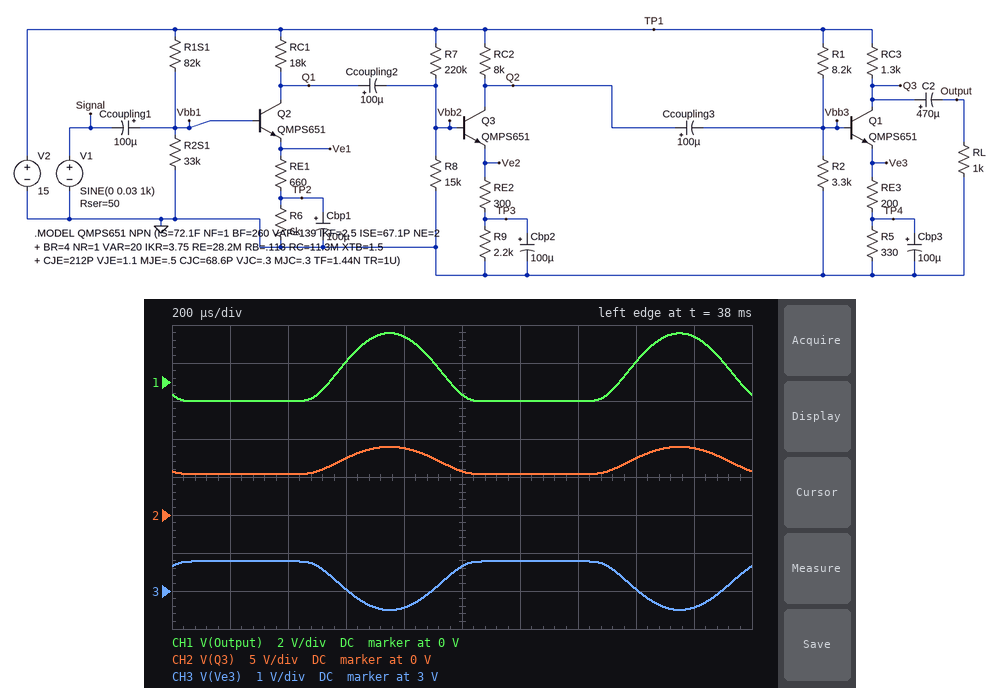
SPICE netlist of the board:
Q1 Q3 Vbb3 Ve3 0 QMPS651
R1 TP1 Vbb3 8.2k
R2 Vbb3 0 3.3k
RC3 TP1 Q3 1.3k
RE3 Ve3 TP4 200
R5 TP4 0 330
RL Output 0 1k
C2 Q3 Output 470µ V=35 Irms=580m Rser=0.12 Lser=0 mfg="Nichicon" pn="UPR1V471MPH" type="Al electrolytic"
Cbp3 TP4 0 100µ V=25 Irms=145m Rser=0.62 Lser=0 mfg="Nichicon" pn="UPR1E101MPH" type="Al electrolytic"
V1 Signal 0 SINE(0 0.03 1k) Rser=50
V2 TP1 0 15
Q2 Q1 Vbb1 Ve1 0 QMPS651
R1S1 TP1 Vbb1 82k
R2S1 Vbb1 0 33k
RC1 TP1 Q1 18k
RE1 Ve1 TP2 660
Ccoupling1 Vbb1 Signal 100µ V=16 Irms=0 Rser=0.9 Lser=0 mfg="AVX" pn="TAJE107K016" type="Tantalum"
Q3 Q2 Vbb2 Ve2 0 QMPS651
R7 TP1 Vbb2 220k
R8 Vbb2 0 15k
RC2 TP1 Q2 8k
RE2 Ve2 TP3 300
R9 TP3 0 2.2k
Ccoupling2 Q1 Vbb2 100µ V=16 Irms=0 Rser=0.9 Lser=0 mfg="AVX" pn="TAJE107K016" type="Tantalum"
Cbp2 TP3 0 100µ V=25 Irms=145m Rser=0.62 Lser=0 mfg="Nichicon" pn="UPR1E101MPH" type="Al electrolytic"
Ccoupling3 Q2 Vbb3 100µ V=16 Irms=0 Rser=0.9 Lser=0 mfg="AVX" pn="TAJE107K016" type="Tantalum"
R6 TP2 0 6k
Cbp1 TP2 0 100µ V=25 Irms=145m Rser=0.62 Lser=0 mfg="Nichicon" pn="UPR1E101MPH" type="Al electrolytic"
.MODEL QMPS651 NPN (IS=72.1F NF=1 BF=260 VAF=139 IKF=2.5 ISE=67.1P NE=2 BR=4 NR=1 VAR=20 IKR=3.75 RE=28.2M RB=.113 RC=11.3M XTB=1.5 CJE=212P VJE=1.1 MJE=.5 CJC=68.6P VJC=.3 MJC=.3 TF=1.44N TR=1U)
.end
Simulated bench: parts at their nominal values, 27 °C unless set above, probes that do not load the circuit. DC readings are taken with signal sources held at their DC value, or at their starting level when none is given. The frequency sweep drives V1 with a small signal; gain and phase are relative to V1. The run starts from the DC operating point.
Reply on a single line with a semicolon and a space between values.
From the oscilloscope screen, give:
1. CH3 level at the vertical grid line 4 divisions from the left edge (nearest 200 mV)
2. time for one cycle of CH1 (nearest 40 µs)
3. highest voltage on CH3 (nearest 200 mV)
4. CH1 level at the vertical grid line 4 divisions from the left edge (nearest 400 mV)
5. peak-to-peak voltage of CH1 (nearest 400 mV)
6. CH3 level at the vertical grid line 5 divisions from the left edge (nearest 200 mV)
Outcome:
2.6 V; 1.00 ms; 3.8 V; 2.4 V; 3.6 V; 3.6 V
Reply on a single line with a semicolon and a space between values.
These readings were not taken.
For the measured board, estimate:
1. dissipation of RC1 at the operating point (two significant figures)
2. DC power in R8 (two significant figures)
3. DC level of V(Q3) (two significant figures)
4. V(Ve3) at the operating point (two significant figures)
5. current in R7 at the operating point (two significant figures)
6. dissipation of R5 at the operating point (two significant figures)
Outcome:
4.9 mW; 55 µW; 6.4 V; 3.5 V; 64 µA; 15 mW
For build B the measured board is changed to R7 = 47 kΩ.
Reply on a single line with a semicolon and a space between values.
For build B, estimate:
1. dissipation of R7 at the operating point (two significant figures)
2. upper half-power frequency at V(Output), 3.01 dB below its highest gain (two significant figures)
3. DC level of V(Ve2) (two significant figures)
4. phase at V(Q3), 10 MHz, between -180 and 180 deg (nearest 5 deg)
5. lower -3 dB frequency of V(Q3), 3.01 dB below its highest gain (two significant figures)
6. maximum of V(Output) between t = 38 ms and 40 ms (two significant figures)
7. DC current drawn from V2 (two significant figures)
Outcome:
2.8 mW; 80 kHz; 2.9 V; -160 deg; 13 Hz; 3.4 V; 10 mA
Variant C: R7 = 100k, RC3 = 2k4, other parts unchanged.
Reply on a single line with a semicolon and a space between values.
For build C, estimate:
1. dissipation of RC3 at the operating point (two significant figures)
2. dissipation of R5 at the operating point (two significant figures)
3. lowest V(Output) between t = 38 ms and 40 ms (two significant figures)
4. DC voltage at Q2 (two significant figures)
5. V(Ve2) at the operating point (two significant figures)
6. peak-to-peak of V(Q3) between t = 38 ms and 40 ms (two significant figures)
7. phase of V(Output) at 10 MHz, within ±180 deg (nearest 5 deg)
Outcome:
61 mW; 9.6 mW; -140 mV; 11 V; 1.3 V; 2.1 V; 135 deg
